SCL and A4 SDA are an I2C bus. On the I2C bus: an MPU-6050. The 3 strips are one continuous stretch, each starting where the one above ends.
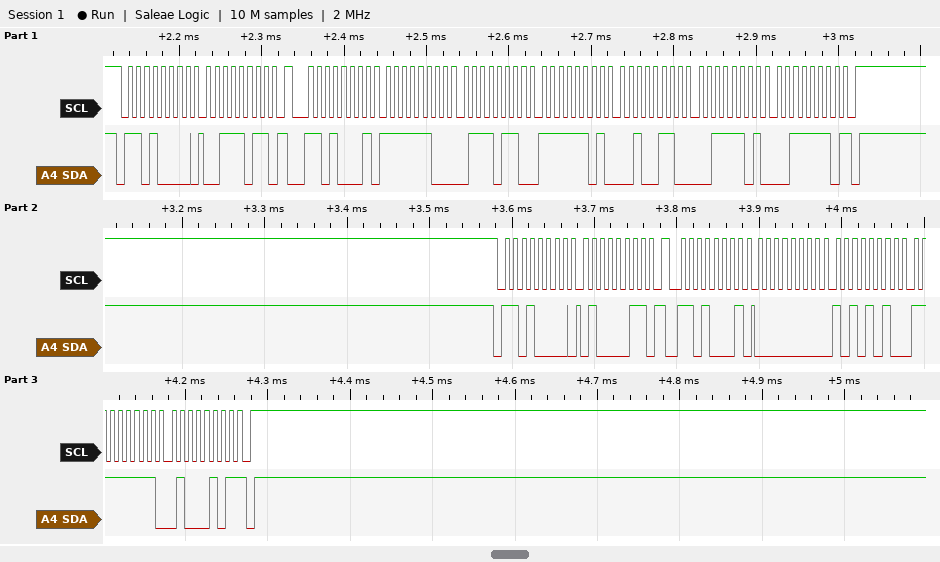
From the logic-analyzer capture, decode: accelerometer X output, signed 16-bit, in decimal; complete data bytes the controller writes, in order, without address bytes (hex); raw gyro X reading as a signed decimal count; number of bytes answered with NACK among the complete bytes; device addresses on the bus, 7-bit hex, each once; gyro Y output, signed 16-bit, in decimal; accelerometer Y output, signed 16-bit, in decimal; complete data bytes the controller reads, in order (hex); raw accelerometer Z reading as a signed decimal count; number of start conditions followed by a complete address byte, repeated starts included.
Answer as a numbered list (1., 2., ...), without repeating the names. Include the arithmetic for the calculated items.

1. 0xFC76 = -906
2. 3B 43
3. 0x00AA = 170
4. 2
5. 0x68
6. 0xFF45 = -187
7. 0xFD26 = -730
8. FC 76 FD 26 3D 3E 00 AA FF 45
9. 0x3D3E = 15678
10. 4
